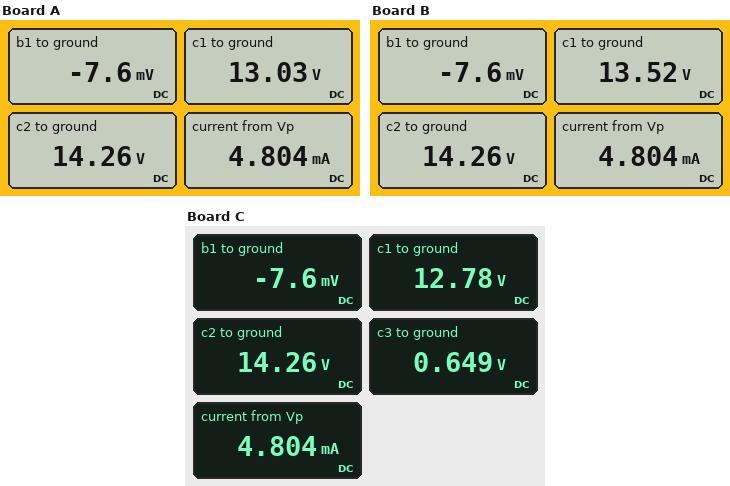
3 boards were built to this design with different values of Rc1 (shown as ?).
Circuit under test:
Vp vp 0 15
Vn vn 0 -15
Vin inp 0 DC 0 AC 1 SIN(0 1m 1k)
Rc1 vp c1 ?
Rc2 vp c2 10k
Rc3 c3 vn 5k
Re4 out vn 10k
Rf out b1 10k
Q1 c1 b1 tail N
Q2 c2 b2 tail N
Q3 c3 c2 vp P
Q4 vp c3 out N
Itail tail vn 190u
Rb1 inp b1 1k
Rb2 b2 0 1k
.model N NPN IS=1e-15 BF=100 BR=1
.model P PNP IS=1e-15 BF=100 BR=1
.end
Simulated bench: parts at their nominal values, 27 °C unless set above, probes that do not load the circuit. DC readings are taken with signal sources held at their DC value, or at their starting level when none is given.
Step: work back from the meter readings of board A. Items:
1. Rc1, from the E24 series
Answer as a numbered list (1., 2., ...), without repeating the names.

1. 24 kΩ
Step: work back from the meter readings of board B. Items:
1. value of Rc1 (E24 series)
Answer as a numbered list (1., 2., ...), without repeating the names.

1. 18 kΩ
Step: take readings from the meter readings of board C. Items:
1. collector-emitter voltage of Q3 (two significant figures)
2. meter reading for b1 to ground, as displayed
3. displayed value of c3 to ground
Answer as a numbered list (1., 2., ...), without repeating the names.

1. -14 V
2. -7.6 mV
3. 0.649 V
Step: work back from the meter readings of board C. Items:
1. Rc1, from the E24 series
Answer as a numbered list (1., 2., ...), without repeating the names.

1. 27 kΩ
